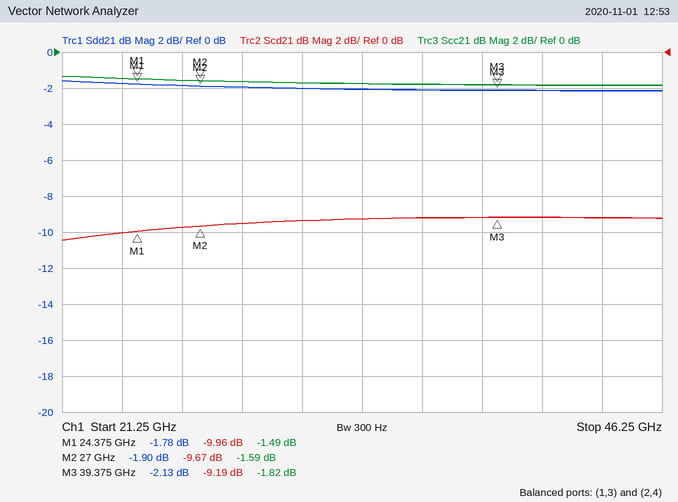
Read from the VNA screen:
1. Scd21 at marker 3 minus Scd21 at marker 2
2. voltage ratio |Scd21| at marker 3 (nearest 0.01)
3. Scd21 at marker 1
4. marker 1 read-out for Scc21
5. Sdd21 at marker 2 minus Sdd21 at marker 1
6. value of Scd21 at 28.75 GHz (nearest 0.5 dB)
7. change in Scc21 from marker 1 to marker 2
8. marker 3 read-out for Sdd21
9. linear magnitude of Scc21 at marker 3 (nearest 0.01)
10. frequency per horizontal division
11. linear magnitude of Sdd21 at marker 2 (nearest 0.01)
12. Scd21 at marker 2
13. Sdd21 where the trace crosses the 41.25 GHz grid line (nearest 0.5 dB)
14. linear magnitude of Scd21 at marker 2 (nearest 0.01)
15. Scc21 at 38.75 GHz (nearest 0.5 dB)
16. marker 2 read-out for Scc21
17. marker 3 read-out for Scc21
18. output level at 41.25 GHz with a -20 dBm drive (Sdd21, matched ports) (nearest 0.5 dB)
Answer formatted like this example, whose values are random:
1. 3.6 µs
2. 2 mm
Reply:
1. 0.48 dB
2. 0.35
3. -9.96 dB
4. -1.49 dB
5. -0.12 dB
6. -9.5 dB
7. -0.10 dB
8. -2.13 dB
9. 0.81
10. 2.5 GHz
11. 0.80
12. -9.67 dB
13. -2.0 dB
14. 0.33
15. -2.0 dB
16. -1.59 dB
17. -1.82 dB
18. -22.0 dBm
